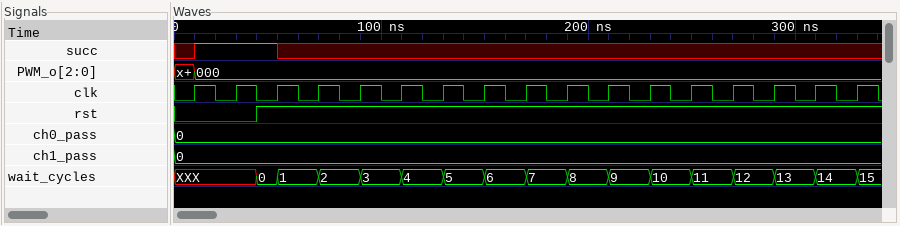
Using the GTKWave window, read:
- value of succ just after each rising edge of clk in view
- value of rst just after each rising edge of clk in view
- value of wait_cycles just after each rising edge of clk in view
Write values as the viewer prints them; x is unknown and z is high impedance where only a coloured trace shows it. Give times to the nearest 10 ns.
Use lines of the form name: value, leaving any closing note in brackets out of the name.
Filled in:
value of succ just after each rising edge of clk in view: 1 1 x x x x x x x x x x x x x x x
value of rst just after each rising edge of clk in view: 0 0 1 1 1 1 1 1 1 1 1 1 1 1 1 1 1
value of wait_cycles just after each rising edge of clk in view: XXX, XXX, 1, 2, 3, 4, 5, 6, 7, 8, 9, 10, 11, 12, 13, 14, 15
